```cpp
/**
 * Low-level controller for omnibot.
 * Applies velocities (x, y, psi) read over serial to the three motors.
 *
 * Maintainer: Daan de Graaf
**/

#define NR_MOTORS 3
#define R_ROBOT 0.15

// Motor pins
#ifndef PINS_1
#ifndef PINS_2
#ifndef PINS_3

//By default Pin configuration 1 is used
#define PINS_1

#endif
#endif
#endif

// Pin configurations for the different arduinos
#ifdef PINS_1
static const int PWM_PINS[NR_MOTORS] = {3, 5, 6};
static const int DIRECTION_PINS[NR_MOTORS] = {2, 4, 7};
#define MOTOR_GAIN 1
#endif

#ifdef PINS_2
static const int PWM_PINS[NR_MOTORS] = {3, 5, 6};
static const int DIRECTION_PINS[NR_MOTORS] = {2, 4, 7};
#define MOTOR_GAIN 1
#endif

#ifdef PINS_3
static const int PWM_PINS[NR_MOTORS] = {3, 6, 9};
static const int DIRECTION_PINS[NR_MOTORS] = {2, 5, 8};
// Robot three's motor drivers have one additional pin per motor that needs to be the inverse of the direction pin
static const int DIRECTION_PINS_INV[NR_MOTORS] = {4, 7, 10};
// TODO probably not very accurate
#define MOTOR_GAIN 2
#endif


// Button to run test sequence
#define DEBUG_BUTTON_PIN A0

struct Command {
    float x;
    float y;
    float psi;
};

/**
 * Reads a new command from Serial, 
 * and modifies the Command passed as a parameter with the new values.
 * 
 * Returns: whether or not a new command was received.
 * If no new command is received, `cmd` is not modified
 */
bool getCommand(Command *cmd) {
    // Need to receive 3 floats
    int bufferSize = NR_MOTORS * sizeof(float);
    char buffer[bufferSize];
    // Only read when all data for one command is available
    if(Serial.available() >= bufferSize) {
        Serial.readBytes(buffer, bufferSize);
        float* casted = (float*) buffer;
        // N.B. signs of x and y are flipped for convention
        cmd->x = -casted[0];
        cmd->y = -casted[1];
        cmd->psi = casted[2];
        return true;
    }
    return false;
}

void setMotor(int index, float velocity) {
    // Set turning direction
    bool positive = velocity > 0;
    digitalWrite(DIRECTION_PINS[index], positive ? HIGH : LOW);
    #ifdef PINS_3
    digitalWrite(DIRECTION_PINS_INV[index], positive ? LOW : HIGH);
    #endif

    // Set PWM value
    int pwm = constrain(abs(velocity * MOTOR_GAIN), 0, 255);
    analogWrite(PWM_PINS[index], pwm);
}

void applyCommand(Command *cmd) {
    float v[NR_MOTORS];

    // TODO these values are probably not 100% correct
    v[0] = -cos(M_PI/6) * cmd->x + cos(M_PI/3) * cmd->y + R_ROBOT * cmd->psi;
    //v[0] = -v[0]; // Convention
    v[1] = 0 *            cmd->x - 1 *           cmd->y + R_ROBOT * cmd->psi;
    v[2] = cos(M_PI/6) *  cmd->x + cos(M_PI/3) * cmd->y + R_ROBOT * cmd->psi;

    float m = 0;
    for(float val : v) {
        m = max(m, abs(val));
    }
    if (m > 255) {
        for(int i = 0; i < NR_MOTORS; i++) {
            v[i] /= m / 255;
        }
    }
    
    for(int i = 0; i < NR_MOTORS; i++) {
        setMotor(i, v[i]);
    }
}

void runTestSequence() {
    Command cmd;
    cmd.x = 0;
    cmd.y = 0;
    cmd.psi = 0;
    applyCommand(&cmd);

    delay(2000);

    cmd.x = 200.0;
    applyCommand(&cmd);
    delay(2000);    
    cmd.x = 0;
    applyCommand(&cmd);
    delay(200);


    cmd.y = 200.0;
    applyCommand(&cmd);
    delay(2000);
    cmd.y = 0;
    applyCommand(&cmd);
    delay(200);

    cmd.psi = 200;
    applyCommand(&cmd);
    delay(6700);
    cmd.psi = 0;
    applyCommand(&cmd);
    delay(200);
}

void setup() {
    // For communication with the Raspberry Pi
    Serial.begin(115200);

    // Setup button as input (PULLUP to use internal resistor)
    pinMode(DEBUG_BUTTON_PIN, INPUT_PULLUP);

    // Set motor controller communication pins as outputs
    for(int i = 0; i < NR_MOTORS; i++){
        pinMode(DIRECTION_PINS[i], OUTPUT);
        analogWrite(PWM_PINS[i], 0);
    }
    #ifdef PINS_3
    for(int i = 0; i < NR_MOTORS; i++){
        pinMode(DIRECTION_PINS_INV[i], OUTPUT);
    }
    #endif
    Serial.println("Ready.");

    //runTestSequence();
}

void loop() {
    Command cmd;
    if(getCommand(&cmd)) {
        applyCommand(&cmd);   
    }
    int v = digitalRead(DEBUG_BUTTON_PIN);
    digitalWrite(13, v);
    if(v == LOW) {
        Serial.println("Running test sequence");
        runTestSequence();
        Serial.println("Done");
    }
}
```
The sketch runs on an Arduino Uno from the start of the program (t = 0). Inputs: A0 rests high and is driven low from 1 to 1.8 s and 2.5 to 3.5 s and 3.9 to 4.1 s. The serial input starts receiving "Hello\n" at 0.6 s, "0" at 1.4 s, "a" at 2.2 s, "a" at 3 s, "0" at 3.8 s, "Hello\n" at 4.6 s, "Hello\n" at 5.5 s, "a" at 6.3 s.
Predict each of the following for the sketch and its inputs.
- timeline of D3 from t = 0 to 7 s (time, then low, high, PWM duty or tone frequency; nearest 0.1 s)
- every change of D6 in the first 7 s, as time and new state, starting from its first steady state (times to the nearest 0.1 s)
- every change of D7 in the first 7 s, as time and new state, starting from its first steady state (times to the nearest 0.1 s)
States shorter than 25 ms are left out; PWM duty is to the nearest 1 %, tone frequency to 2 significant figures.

0 s low; 3 s PWM 68 %; 5 s low; 5.2 s PWM 39 %
0 s low; 3 s PWM 68 %; 5 s low; 5.2 s PWM 39 %
0 s low; 3 s high; 5 s low; 5.2 s high
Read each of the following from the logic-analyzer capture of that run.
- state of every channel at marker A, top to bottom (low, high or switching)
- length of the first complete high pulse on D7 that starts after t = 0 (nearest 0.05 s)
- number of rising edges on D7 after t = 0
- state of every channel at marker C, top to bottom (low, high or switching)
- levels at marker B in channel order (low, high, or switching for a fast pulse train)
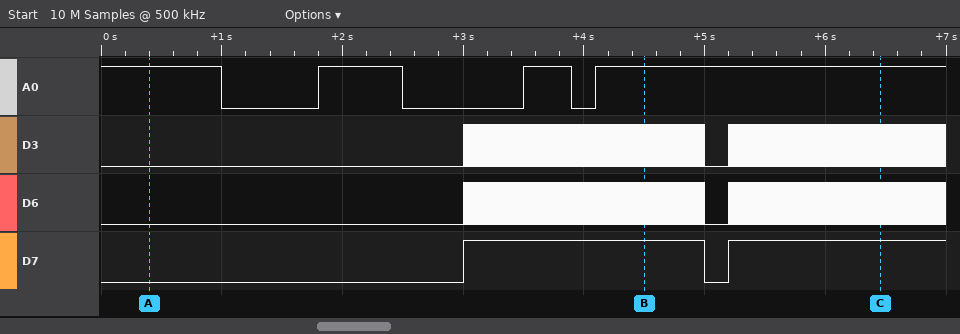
A0 high, D3 low, D6 low, D7 low
2.00 s
2
A0 high, D3 switching, D6 switching, D7 high
A0 high, D3 switching, D6 switching, D7 high
